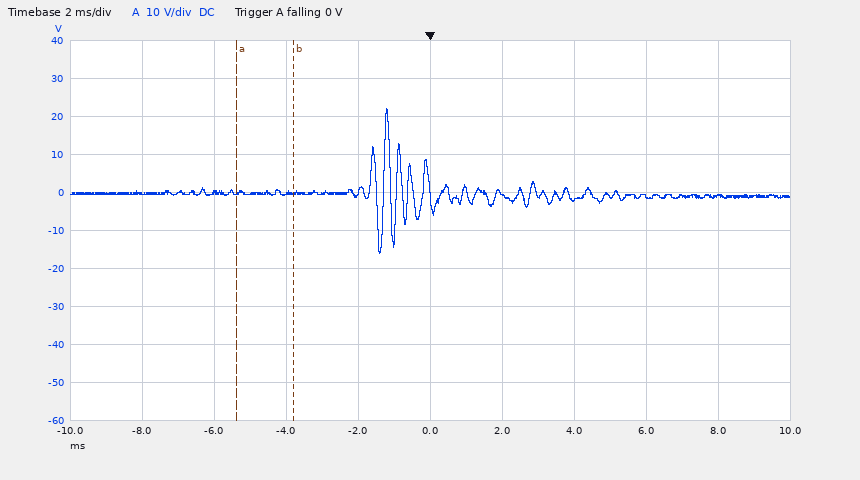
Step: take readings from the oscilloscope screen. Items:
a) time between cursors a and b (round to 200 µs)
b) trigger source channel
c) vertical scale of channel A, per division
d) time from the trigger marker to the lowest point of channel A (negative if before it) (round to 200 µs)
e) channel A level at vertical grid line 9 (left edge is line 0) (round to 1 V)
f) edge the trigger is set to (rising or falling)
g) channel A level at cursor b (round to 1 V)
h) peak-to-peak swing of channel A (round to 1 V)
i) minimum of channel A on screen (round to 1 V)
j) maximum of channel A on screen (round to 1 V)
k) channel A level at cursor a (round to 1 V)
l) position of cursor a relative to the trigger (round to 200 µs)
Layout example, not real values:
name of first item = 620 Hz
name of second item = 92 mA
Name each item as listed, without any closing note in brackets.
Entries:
time between cursors a and b = 1.6 ms
trigger source channel = channel A
vertical scale of channel A, per division = 10 V
time from the trigger marker to the lowest point of channel A (negative if before it) = -1.4 ms
channel A level at vertical grid line 9 (left edge is line 0) = -1 V
edge the trigger is set to = falling
channel A level at cursor b = 0 V
peak-to-peak swing of channel A = 38 V
minimum of channel A on screen = -16 V
maximum of channel A on screen = 22 V
channel A level at cursor a = 0 V
position of cursor a relative to the trigger = -5.4 ms
